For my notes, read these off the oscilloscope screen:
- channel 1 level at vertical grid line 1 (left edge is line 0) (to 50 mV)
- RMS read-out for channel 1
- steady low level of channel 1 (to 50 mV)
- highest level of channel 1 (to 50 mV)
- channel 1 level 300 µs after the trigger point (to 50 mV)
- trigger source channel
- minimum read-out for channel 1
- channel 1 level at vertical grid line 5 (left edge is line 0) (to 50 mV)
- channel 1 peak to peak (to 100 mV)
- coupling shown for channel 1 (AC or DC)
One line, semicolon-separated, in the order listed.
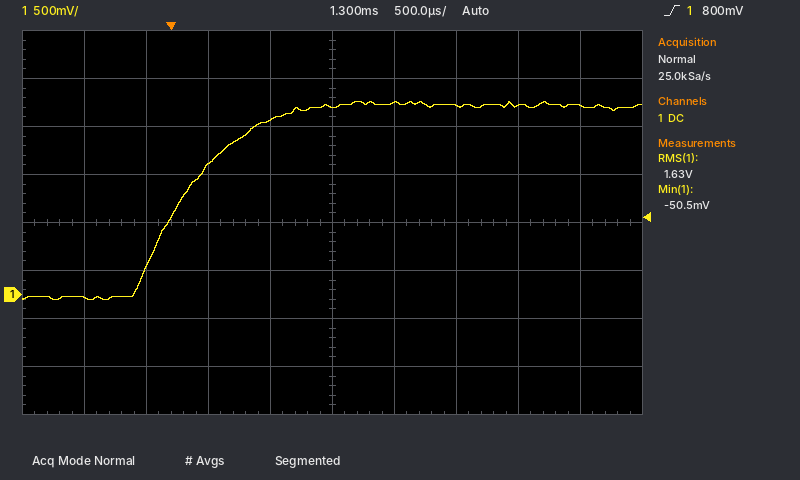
-50 mV; 1.63 V; 0 mV; 2.00 V; 1.35 V; channel 1; -50.5 mV; 1.95 V; 2.10 V; DC
